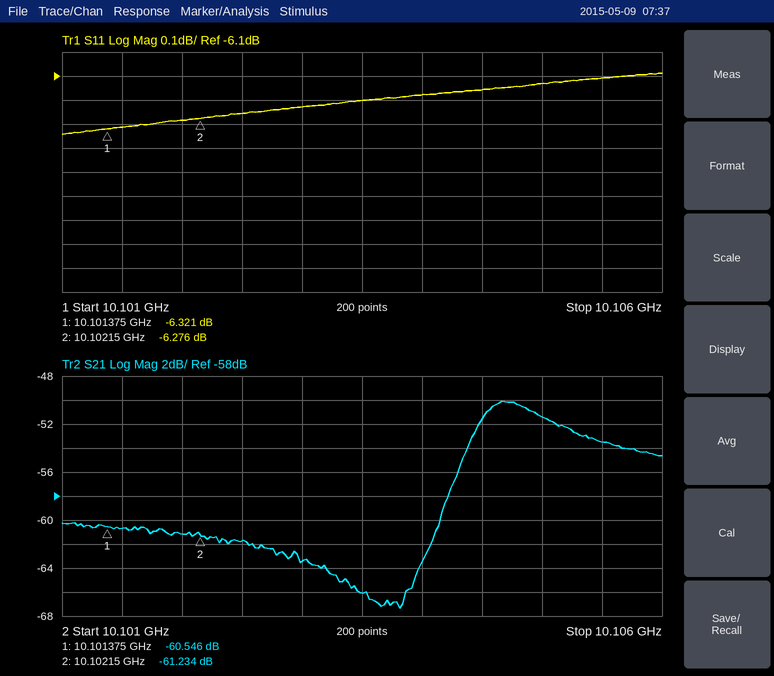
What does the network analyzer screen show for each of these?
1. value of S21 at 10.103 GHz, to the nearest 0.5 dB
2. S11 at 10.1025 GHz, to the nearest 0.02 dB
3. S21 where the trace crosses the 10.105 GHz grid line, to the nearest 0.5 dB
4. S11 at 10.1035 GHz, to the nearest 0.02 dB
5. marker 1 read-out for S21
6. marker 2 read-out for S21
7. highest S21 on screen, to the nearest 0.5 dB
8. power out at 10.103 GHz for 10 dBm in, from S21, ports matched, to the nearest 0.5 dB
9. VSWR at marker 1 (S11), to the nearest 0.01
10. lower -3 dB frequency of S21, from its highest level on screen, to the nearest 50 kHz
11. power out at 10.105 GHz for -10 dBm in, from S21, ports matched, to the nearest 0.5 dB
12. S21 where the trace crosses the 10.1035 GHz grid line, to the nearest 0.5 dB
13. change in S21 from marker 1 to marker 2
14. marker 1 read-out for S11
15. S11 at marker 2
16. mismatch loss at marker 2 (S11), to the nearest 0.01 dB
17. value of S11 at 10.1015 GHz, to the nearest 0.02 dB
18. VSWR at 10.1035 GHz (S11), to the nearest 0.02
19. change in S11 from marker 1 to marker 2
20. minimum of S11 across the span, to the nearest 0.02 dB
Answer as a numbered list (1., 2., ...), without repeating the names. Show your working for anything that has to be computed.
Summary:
1. -63.5 dB
2. -6.26 dB
3. -51.5 dB
4. -6.20 dB
5. -60.546 dB
6. -61.234 dB
7. -50.0 dB
8. 10 dBm + (-63.5 dB) = -53.5 dBm
9. (1 + 0.4830)/(1 − 0.4830) ≈ 2.87
10. 10.10440 GHz
11. -10 dBm + (-51.5 dB) = -61.5 dBm
12. -66.0 dB
13. -61.234 − (-60.546) = -0.688 dB
14. -6.321 dB
15. -6.276 dB
16. −10 log10(1 − 10^(-6.276/10)) ≈ 1.17 dB
17. -6.32 dB
18. |Γ| = 10^(-6.2/20) = 0.4898; VSWR = (1 + 0.4898)/(1 − 0.4898) ≈ 2.92
19. -6.276 − (-6.321) = 0.045 dB
20. -6.34 dB
